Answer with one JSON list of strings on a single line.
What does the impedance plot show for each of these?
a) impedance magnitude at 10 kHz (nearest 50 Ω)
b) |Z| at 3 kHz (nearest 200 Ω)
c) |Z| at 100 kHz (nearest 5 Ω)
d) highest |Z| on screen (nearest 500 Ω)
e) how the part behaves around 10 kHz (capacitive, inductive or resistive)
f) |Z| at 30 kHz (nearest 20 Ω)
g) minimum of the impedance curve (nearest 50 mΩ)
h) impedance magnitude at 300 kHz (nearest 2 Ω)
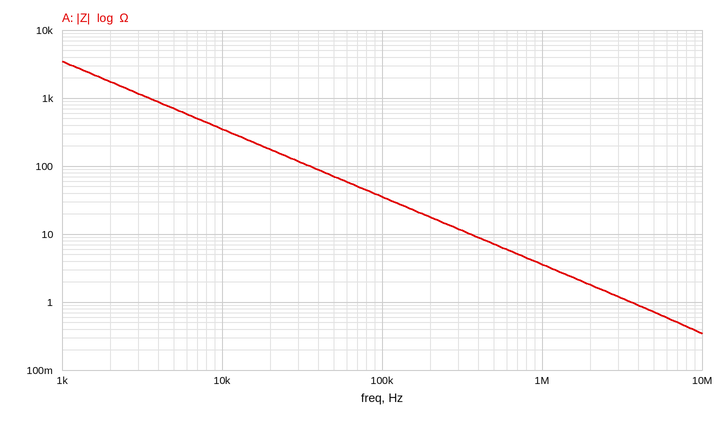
["350 Ω", "1.2 kΩ", "35 Ω", "3.5 kΩ", "capacitive", "120 Ω", "350 mΩ", "12 Ω"]
